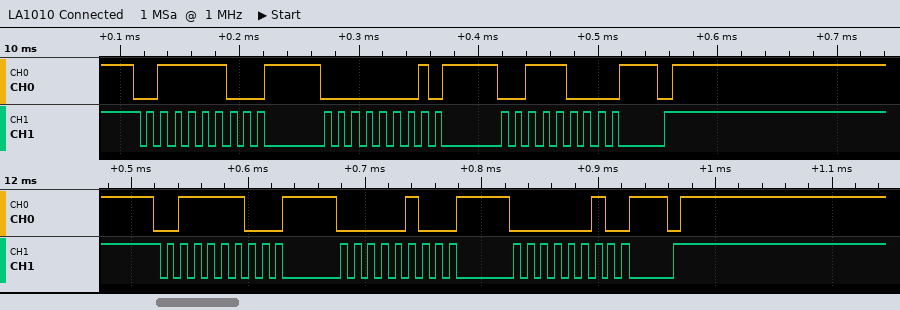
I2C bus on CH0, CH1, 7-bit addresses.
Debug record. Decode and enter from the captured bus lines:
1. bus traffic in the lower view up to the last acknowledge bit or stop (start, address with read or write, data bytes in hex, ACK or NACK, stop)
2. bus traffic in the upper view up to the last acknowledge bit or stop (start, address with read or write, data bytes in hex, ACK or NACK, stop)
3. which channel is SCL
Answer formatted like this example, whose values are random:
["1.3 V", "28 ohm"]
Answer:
["start, address 3E write ACK, 04 ACK, 02 ACK, stop", "start, address 3E write ACK, 01 ACK, 38 ACK, stop", "CH1"]
